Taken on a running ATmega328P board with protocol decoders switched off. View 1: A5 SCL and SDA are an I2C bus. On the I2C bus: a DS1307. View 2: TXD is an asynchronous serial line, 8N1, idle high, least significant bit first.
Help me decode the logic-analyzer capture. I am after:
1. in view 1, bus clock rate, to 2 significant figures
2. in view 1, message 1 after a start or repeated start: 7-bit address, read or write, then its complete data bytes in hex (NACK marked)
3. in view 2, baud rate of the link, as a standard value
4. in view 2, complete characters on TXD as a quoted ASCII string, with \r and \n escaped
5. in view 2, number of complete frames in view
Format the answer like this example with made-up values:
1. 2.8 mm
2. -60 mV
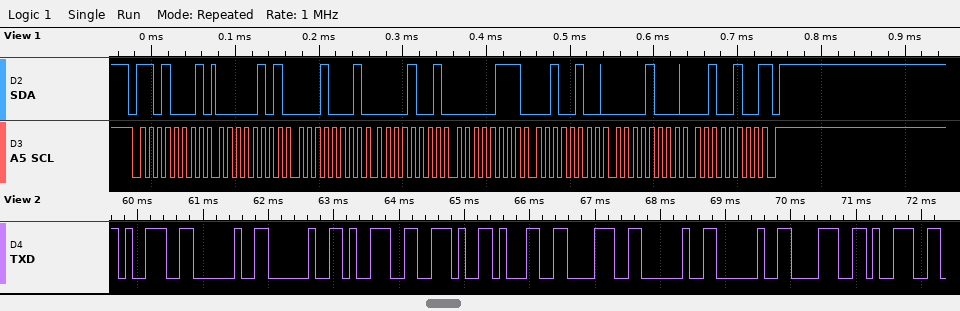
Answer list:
1. 100 kHz
2. 0x68 read: 05 11 09 07 24 08 24 NACK
3. 9600 baud
4. "9  9.18  89"
5. 11
